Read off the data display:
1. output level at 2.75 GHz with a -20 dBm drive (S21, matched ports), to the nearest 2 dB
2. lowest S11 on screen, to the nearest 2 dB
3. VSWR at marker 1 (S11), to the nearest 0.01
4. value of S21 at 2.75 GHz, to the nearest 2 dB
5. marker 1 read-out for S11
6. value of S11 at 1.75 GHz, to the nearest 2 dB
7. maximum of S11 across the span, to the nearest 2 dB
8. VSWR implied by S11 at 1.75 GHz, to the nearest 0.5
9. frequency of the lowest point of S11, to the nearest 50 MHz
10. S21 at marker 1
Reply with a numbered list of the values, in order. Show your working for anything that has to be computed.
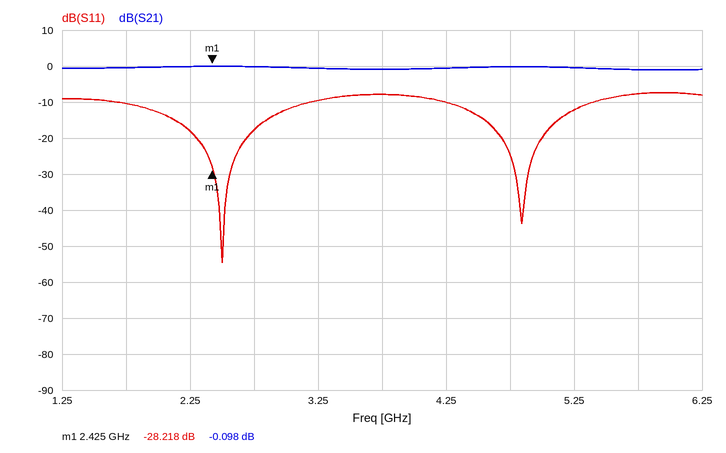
1. -20 dBm + (0 dB) = -20 dBm
2. -54 dB
3. (1 + 0.0388)/(1 − 0.0388) ≈ 1.08
4. 0 dB
5. -28.218 dB
6. -10 dB
7. -8 dB
8. |Γ| = 10^(-10/20) = 0.3162; VSWR = (1 + 0.3162)/(1 − 0.3162) ≈ 1.92, so 2.0 to the nearest 0.5
9. 2.50 GHz
10. -0.098 dB
